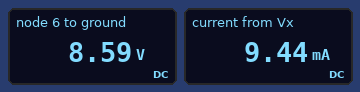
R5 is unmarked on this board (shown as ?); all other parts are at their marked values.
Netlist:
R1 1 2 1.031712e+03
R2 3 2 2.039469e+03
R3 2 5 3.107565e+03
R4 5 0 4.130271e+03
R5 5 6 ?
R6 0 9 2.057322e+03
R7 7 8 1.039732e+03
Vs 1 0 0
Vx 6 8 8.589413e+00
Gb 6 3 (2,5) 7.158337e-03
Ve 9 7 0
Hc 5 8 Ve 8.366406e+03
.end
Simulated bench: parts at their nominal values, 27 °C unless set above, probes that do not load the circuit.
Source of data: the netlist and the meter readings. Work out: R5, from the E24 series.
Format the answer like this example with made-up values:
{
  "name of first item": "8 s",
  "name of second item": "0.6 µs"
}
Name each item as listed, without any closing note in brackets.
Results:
{
  "R5, from the E24 series": "910 Ω"
}
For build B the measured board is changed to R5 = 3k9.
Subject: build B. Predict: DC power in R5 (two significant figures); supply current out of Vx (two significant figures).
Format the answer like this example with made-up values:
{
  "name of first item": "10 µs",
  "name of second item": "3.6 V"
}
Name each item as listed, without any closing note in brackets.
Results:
{
  "DC power in R5": "19 mW",
  "supply current out of Vx": "2.2 mA"
}
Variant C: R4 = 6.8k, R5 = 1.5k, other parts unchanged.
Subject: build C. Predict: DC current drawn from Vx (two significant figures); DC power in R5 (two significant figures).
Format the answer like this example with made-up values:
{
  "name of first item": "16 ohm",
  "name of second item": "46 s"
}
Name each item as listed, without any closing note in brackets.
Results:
{
  "DC current drawn from Vx": "5.7 mA",
  "DC power in R5": "49 mW"
}
